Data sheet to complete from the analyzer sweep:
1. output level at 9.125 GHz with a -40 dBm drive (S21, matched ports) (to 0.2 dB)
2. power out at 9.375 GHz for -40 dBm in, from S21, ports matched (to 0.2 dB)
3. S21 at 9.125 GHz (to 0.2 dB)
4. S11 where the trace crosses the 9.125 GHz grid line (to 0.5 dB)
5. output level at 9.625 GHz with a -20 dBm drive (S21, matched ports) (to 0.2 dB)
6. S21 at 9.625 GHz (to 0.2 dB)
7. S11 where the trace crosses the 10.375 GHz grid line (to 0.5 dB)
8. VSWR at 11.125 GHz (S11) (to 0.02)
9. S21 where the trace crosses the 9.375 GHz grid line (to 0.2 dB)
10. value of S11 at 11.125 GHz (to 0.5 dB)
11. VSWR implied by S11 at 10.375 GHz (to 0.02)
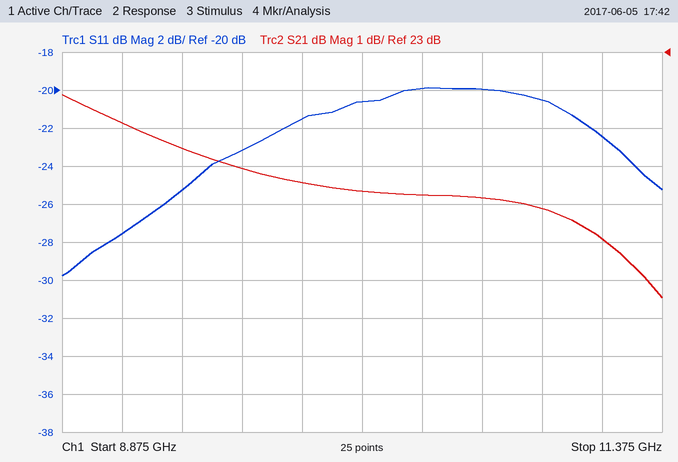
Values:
-18.8 dBm
-19.6 dBm
21.2 dB
-27.5 dB
0.0 dBm
20.0 dB
-20.0 dB
1.16
20.4 dB
-22.5 dB
1.22
